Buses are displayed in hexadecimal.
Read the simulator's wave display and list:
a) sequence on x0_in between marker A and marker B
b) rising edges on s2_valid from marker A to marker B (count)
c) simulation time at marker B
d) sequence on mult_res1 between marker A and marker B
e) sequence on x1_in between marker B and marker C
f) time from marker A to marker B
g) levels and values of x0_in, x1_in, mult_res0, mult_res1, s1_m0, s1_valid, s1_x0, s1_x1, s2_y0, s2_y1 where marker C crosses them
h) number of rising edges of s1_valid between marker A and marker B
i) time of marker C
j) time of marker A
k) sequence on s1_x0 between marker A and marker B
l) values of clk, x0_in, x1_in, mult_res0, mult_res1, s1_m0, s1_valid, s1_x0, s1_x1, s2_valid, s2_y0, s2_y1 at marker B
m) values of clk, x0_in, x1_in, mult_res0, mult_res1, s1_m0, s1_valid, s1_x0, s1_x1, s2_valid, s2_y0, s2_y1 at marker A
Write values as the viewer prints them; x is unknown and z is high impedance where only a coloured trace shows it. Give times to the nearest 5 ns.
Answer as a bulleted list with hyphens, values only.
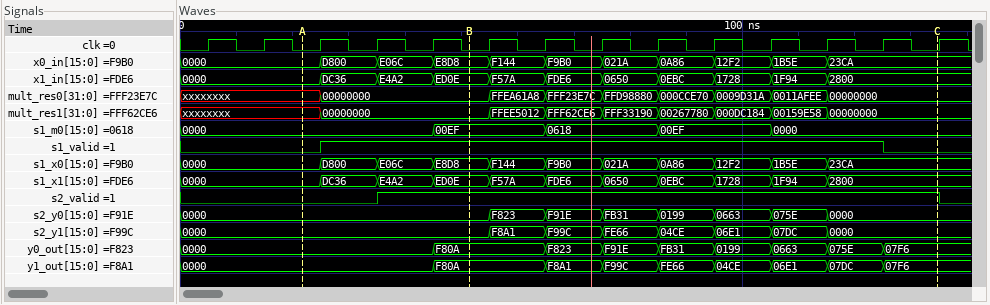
- 0000, D800, E06C, E8D8
- 1
- 50 ns
- xxxxxxxx, 00000000
- ED0E, F57A, FDE6, 0650, 0EBC, 1728, 1F94, 2800
- 30 ns
- x0_in=23CA, x1_in=2800, mult_res0=00000000, mult_res1=00000000, s1_m0=0000, s1_valid=0, s1_x0=23CA, s1_x1=2800, s2_y0=0000, s2_y1=0000
- 1
- 135 ns
- 20 ns
- 0000, D800, E06C, E8D8
- clk=0, x0_in=E8D8, x1_in=ED0E, mult_res0=00000000, mult_res1=00000000, s1_m0=00EF, s1_valid=1, s1_x0=E8D8, s1_x1=ED0E, s2_valid=1, s2_y0=0000, s2_y1=0000
- clk=0, x0_in=0000, x1_in=0000, mult_res0=xxxxxxxx, mult_res1=xxxxxxxx, s1_m0=0000, s1_valid=0, s1_x0=0000, s1_x1=0000, s2_valid=0, s2_y0=0000, s2_y1=0000
